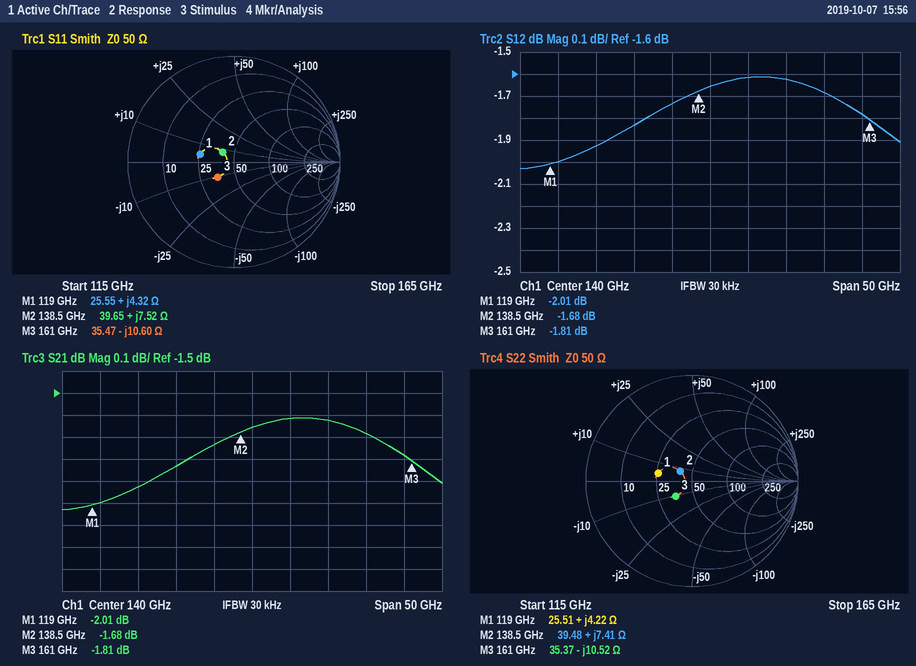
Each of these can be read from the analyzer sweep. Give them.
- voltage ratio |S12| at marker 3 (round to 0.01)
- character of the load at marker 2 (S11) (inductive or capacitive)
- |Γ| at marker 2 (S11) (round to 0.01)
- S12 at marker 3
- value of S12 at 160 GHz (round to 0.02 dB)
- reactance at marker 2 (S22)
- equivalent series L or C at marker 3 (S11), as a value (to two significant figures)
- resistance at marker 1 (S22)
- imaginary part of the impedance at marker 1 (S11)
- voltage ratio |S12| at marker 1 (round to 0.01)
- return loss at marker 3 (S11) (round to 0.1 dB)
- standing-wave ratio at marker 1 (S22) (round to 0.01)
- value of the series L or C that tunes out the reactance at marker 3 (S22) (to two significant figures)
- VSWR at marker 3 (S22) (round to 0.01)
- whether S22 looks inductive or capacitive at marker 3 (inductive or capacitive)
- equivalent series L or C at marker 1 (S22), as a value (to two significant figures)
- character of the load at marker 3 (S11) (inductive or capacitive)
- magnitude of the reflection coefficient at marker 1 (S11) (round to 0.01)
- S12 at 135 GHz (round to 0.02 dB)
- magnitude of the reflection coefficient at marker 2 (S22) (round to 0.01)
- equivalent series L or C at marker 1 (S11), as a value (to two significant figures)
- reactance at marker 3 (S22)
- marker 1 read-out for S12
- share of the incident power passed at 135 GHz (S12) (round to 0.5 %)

0.81
inductive
0.14
-1.81 dB
-1.78 dB
+7.41 Ω
93 fF
25.51 Ω
+4.32 Ω
0.79
13.6 dB
1.98
10 pH
1.53
capacitive
5.6 pH
capacitive
0.33
-1.74 dB
0.14
5.8 pH
-10.52 Ω
-2.01 dB
67.0 %
